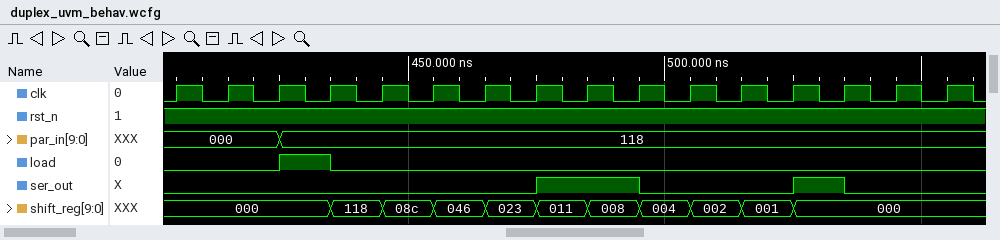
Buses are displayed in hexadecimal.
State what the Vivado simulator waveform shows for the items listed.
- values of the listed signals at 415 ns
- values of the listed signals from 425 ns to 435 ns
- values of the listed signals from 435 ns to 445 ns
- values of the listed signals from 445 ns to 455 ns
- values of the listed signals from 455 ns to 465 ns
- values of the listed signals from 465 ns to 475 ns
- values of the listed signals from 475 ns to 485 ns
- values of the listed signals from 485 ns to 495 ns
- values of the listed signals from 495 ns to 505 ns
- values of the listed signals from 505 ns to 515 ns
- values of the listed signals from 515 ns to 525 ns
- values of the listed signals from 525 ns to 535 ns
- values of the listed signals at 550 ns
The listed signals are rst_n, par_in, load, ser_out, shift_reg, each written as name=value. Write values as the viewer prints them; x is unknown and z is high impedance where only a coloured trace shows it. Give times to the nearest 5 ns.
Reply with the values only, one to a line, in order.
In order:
rst_n=1, par_in=000, load=0, ser_out=0, shift_reg=000
rst_n=1, par_in=118, load=1, ser_out=0, shift_reg=000
rst_n=1, par_in=118, load=0, ser_out=0, shift_reg=118
rst_n=1, par_in=118, load=0, ser_out=0, shift_reg=08c
rst_n=1, par_in=118, load=0, ser_out=0, shift_reg=046
rst_n=1, par_in=118, load=0, ser_out=0, shift_reg=023
rst_n=1, par_in=118, load=0, ser_out=1, shift_reg=011
rst_n=1, par_in=118, load=0, ser_out=1, shift_reg=008
rst_n=1, par_in=118, load=0, ser_out=0, shift_reg=004
rst_n=1, par_in=118, load=0, ser_out=0, shift_reg=002
rst_n=1, par_in=118, load=0, ser_out=0, shift_reg=001
rst_n=1, par_in=118, load=0, ser_out=1, shift_reg=000
rst_n=1, par_in=118, load=0, ser_out=0, shift_reg=000
